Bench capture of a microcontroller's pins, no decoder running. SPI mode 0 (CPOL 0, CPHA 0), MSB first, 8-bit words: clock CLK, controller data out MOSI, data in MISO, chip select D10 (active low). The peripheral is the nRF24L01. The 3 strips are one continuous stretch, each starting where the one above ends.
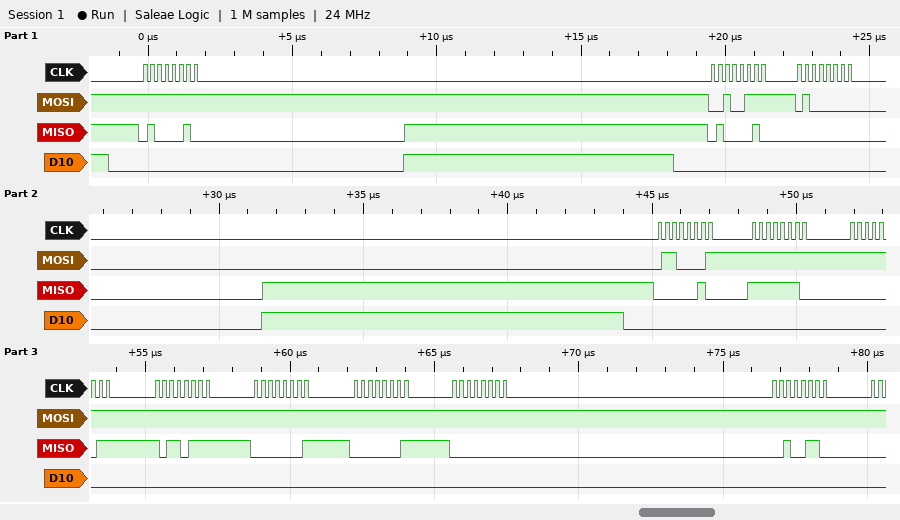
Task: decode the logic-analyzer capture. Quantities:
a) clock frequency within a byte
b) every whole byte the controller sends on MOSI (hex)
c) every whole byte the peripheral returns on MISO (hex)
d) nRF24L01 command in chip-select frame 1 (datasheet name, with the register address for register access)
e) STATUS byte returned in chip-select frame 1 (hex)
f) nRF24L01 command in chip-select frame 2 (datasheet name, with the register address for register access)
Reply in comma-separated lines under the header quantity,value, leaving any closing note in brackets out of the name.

quantity,value
clock frequency within a byte,4 MHz
every whole byte the controller sends on MOSI,0xFF 0x27 0x40 0x61 0xFF 0xFF 0xFF 0xFF 0xFF 0xFF 0xFF
every whole byte the peripheral returns on MISO,0x42 0x42 0x00 0x02 0xFE 0x03 0xB7 0x01 0x01 0x00 0x26
nRF24L01 command in chip-select frame 1,NOP
STATUS byte returned in chip-select frame 1,0x42
nRF24L01 command in chip-select frame 2,W_REGISTER 0x07
